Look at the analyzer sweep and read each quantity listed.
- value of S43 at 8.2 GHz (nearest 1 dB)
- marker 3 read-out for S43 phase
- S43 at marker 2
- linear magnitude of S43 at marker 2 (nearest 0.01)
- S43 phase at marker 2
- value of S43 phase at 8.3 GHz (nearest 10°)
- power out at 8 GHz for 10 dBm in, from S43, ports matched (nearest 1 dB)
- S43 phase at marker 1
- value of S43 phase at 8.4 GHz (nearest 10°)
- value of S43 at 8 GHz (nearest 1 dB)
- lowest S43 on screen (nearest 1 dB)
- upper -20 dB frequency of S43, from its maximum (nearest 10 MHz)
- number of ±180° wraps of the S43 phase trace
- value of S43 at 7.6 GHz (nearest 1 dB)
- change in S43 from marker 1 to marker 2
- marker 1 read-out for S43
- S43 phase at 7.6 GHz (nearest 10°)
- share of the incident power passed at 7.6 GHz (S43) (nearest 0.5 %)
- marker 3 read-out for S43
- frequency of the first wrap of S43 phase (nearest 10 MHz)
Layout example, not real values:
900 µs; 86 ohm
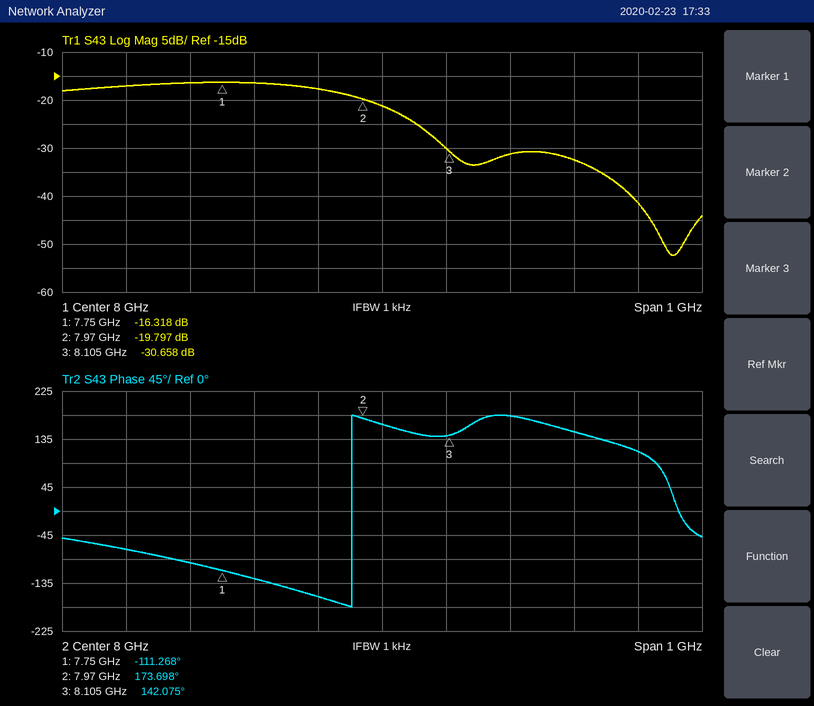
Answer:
-31 dB; 142.075°; -19.797 dB; 0.10; 173.698°; 150°; -11 dBm; -111.268°; 110°; -21 dB; -52 dB; 8.36 GHz; 1; -17 dB; -3.479 dB; -16.318 dB; -70°; 2.0 %; -30.658 dB; 7.95 GHz
